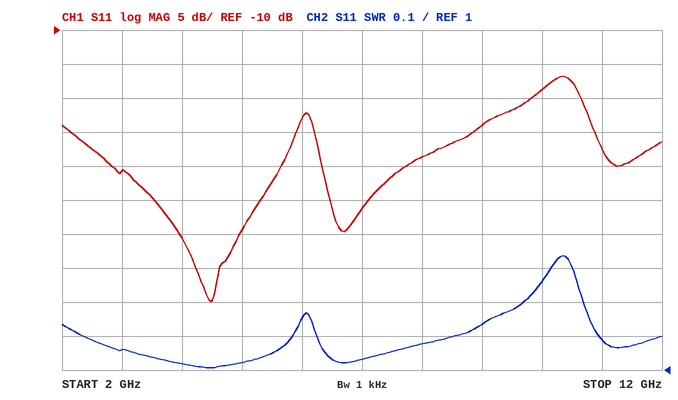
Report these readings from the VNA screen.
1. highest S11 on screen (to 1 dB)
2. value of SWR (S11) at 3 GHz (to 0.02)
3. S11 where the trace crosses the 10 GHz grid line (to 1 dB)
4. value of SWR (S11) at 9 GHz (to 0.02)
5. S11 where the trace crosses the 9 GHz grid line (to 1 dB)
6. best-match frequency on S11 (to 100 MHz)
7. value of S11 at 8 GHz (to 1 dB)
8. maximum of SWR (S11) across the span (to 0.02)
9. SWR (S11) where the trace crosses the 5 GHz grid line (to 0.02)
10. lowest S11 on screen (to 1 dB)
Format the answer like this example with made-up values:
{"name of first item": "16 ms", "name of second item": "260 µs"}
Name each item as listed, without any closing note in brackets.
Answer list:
{"highest S11 on screen": "-17 dB", "value of SWR (S11) at 3 GHz": "1.06", "S11 where the trace crosses the 10 GHz grid line": "-19 dB", "value of SWR (S11) at 9 GHz": "1.14", "S11 where the trace crosses the 9 GHz grid line": "-24 dB", "best-match frequency on S11": "4.5 GHz", "value of S11 at 8 GHz": "-29 dB", "maximum of SWR (S11) across the span": "1.34", "SWR (S11) where the trace crosses the 5 GHz grid line": "1.02", "lowest S11 on screen": "-50 dB"}
